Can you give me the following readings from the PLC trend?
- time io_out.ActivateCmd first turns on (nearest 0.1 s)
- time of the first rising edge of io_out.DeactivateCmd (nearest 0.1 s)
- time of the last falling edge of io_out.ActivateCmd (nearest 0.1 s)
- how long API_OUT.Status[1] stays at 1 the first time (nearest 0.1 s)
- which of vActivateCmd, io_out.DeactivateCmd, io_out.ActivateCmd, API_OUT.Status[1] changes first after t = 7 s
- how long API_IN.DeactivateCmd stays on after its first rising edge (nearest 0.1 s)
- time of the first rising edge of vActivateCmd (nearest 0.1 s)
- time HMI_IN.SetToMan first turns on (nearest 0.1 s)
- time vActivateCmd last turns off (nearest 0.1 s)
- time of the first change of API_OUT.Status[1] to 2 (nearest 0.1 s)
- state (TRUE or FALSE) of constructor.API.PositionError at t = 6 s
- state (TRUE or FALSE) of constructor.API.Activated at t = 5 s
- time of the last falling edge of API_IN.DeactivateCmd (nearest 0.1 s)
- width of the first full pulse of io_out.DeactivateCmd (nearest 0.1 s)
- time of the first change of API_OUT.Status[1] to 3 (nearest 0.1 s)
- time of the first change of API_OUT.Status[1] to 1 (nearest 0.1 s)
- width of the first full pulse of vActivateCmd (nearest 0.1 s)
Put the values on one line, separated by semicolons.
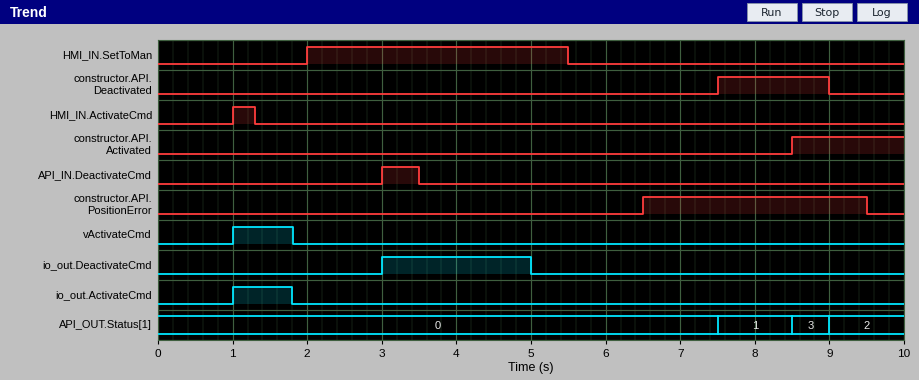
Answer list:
1.0 s; 3.0 s; 1.8 s; 1.0 s; API_OUT.Status[1]; 0.5 s; 1.0 s; 2.0 s; 1.8 s; 9.0 s; FALSE; FALSE; 3.5 s; 2.0 s; 8.5 s; 7.5 s; 0.8 s
